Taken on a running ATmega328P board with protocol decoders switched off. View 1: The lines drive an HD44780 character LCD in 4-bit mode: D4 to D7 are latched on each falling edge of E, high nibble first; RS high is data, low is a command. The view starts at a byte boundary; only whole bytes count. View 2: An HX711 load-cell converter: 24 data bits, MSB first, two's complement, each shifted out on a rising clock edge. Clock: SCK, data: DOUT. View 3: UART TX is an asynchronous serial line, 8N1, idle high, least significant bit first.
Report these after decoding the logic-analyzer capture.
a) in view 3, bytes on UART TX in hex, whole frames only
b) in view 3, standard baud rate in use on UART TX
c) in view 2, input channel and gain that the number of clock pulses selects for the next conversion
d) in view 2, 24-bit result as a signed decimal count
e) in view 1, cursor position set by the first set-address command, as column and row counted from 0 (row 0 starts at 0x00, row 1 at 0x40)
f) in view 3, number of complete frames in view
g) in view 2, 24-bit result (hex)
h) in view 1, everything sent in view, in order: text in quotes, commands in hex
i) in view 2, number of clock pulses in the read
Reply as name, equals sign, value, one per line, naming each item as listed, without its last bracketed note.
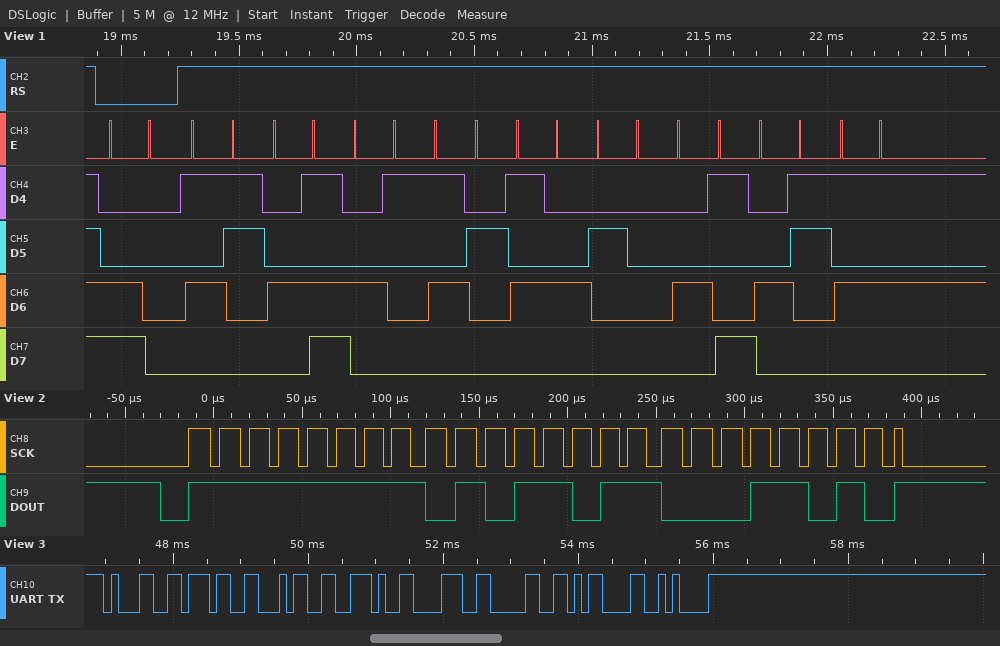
in view 3, bytes on UART TX in hex, whole frames only = 0x31 0x37 0x34 0x2E 0x38 0x30 0x0D 0x0A
in view 3, standard baud rate in use on UART TX = 9600 baud
in view 2, input channel and gain that the number of clock pulses selects for the next conversion = channel A, gain 128
in view 2, 24-bit result as a signed decimal count = -42214
in view 1, cursor position set by the first set-address command, as column and row counted from 0 = column 0, row 1
in view 3, number of complete frames in view = 8
in view 2, 24-bit result = 0xFF5B1A
in view 1, everything sent in view, in order: text in quotes, commands in hex = 0xC0 "SMART ICU"
in view 2, number of clock pulses in the read = 25
